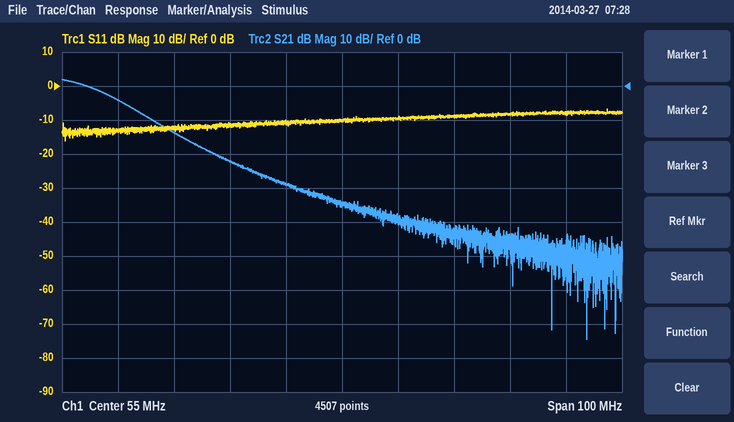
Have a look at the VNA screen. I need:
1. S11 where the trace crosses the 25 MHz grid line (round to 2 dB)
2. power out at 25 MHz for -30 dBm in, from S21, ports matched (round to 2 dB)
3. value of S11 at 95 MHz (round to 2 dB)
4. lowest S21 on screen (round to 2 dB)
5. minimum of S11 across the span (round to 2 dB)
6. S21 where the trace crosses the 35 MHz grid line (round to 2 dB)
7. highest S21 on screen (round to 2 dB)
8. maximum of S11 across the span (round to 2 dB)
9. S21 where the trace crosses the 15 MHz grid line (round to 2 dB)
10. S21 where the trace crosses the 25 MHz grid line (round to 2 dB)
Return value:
-12 dB
-44 dBm
-8 dB
-74 dB
-16 dB
-22 dB
2 dB
-6 dB
-4 dB
-14 dB
